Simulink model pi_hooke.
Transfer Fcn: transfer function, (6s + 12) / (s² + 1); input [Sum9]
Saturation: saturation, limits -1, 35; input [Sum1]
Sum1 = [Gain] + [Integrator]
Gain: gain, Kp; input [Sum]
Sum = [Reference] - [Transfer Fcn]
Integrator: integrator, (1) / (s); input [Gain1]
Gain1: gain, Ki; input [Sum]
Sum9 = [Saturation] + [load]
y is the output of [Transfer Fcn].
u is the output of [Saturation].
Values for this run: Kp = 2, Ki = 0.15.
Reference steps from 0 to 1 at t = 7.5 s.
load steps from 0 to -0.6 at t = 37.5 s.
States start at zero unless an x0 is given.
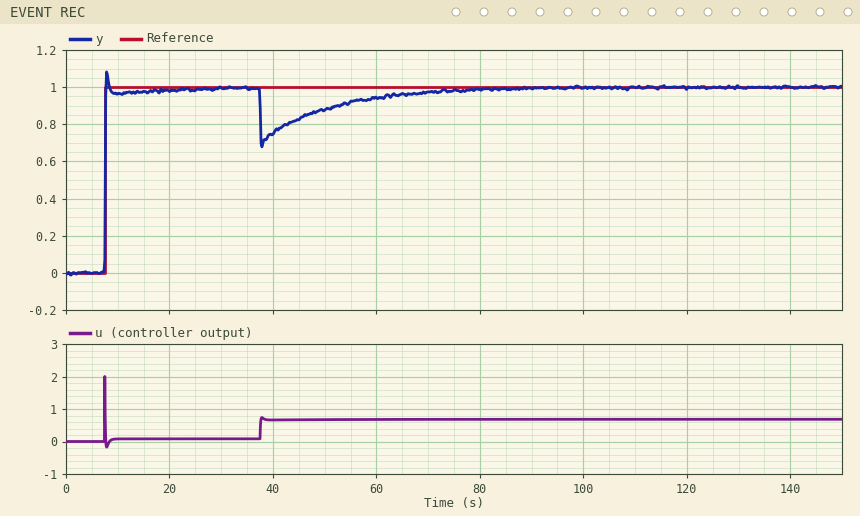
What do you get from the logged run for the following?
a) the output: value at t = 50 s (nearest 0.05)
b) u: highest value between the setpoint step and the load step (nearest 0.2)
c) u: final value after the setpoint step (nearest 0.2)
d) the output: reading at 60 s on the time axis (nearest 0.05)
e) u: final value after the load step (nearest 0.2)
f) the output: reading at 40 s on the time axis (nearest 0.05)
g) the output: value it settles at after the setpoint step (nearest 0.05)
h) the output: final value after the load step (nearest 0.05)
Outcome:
0.90
2.0
0.0
0.95
0.6
0.75
1.00
1.00
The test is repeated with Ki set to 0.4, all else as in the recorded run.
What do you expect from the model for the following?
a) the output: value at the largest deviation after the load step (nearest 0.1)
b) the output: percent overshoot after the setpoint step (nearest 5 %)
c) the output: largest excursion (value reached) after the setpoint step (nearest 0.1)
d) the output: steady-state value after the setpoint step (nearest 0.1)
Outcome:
0.7
10 %
1.1
1.0
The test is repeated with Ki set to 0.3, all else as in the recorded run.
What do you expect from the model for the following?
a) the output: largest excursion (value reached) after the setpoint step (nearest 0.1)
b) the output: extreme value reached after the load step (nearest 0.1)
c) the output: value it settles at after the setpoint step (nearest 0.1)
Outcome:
1.1
0.7
1.0
